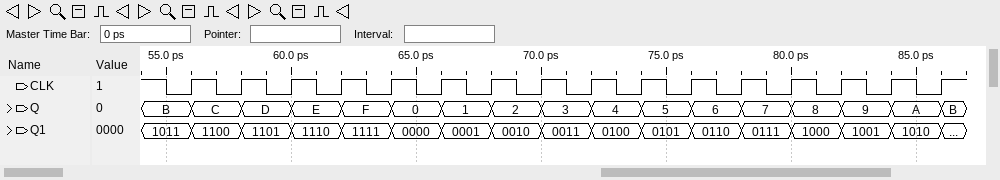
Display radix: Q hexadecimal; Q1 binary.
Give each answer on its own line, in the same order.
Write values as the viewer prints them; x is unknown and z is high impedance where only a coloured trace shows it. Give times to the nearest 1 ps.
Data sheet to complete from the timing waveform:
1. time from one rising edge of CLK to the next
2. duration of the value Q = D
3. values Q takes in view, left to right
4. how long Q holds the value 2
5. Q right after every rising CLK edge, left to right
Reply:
2 ps
2 ps
B, C, D, E, F, 0, 1, 2, 3, 4, 5, 6, 7, 8, 9, A, B
2 ps
C, D, E, F, 0, 1, 2, 3, 4, 5, 6, 7, 8, 9, A, B
